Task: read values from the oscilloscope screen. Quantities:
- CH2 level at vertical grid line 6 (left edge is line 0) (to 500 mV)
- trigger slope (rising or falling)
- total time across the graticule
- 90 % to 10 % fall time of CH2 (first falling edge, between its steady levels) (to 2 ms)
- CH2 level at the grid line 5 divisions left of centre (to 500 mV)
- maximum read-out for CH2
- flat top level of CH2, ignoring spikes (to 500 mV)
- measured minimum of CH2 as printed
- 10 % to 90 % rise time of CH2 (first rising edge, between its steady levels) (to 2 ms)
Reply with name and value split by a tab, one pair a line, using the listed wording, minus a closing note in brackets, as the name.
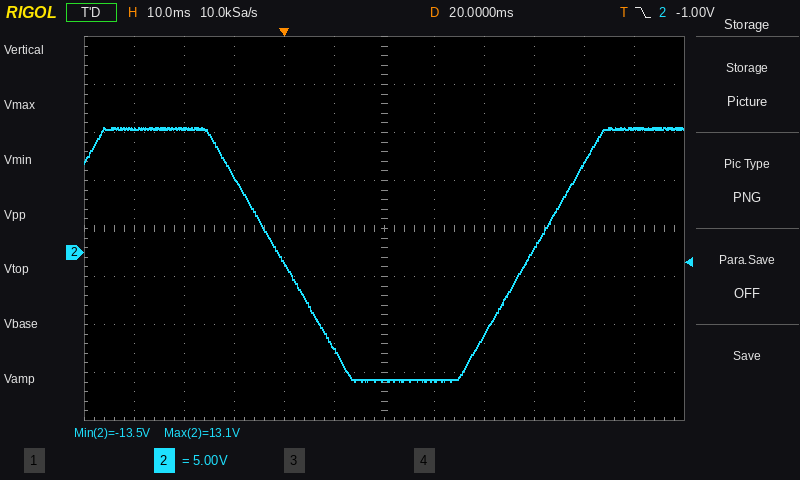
CH2 level at vertical grid line 6 (left edge is line 0)	-13.5 V
trigger slope	falling
total time across the graticule	120 ms
90 % to 10 % fall time of CH2 (first falling edge, between its steady levels)	24 ms
CH2 level at the grid line 5 divisions left of centre	13.0 V
maximum read-out for CH2	13.1 V
flat top level of CH2, ignoring spikes	13.0 V
measured minimum of CH2 as printed	-13.5 V
10 % to 90 % rise time of CH2 (first rising edge, between its steady levels)	24 ms
